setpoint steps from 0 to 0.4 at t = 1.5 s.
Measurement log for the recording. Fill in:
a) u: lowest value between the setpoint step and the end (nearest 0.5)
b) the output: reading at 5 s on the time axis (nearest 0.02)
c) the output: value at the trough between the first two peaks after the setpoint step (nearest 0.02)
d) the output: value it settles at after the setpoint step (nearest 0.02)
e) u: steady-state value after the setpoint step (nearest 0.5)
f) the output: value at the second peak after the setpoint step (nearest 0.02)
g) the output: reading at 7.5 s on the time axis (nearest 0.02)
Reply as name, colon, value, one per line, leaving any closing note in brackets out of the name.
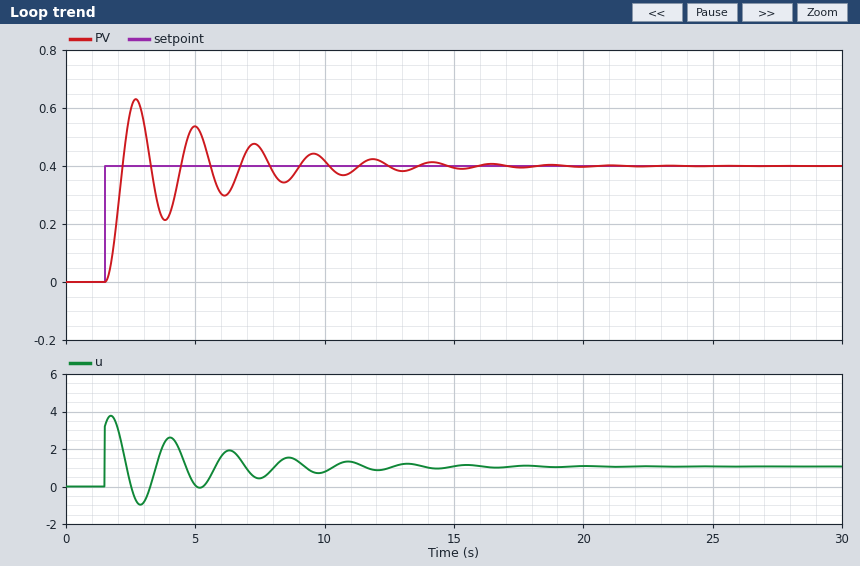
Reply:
u: lowest value between the setpoint step and the end: -1.0
the output: reading at 5 s on the time axis: 0.54
the output: value at the trough between the first two peaks after the setpoint step: 0.22
the output: value it settles at after the setpoint step: 0.40
u: steady-state value after the setpoint step: 1.0
the output: value at the second peak after the setpoint step: 0.54
the output: reading at 7.5 s on the time axis: 0.46
